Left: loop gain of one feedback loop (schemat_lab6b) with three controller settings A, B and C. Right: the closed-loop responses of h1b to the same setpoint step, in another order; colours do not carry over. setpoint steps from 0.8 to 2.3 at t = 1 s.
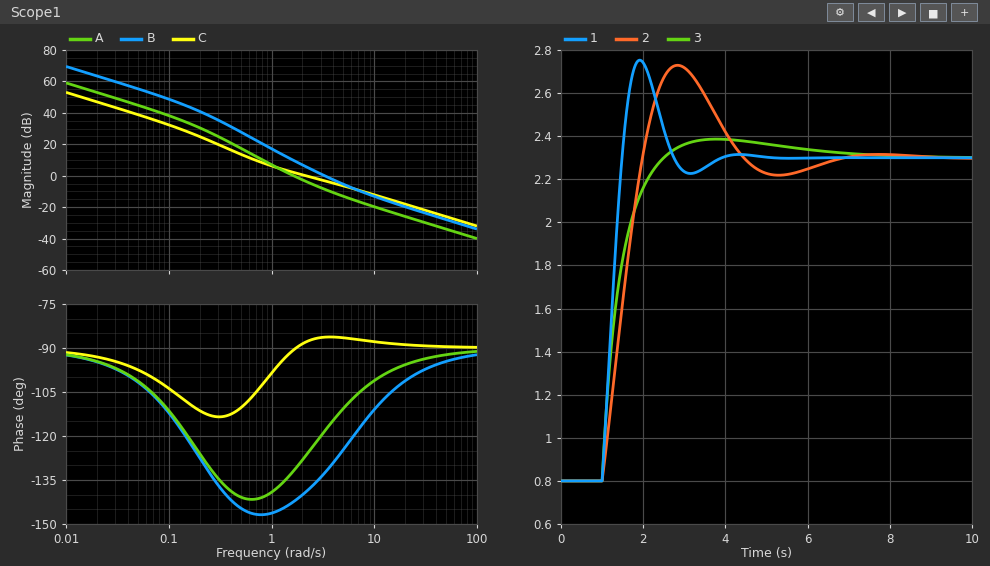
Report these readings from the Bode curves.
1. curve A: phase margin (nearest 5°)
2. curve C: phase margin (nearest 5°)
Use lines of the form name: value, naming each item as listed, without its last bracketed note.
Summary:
curve A: phase margin: 50°
curve C: phase margin: 90°
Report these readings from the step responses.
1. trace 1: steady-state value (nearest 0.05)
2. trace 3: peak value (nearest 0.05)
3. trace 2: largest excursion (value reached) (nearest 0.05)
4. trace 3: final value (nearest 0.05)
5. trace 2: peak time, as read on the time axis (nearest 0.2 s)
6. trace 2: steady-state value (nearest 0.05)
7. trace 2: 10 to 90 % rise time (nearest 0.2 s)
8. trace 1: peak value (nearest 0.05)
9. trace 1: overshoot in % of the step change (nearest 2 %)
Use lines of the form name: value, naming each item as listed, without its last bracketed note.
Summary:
trace 1: steady-state value: 2.30
trace 3: peak value: 2.40
trace 2: largest excursion (value reached): 2.75
trace 3: final value: 2.30
trace 2: peak time, as read on the time axis: 2.8 s
trace 2: steady-state value: 2.30
trace 2: 10 to 90 % rise time: 0.8 s
trace 1: peak value: 2.75
trace 1: overshoot in % of the step change: 30 %
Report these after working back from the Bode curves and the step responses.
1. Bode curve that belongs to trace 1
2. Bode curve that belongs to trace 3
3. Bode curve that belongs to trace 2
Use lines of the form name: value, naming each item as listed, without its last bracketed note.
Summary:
Bode curve that belongs to trace 1: B
Bode curve that belongs to trace 3: C
Bode curve that belongs to trace 2: A
